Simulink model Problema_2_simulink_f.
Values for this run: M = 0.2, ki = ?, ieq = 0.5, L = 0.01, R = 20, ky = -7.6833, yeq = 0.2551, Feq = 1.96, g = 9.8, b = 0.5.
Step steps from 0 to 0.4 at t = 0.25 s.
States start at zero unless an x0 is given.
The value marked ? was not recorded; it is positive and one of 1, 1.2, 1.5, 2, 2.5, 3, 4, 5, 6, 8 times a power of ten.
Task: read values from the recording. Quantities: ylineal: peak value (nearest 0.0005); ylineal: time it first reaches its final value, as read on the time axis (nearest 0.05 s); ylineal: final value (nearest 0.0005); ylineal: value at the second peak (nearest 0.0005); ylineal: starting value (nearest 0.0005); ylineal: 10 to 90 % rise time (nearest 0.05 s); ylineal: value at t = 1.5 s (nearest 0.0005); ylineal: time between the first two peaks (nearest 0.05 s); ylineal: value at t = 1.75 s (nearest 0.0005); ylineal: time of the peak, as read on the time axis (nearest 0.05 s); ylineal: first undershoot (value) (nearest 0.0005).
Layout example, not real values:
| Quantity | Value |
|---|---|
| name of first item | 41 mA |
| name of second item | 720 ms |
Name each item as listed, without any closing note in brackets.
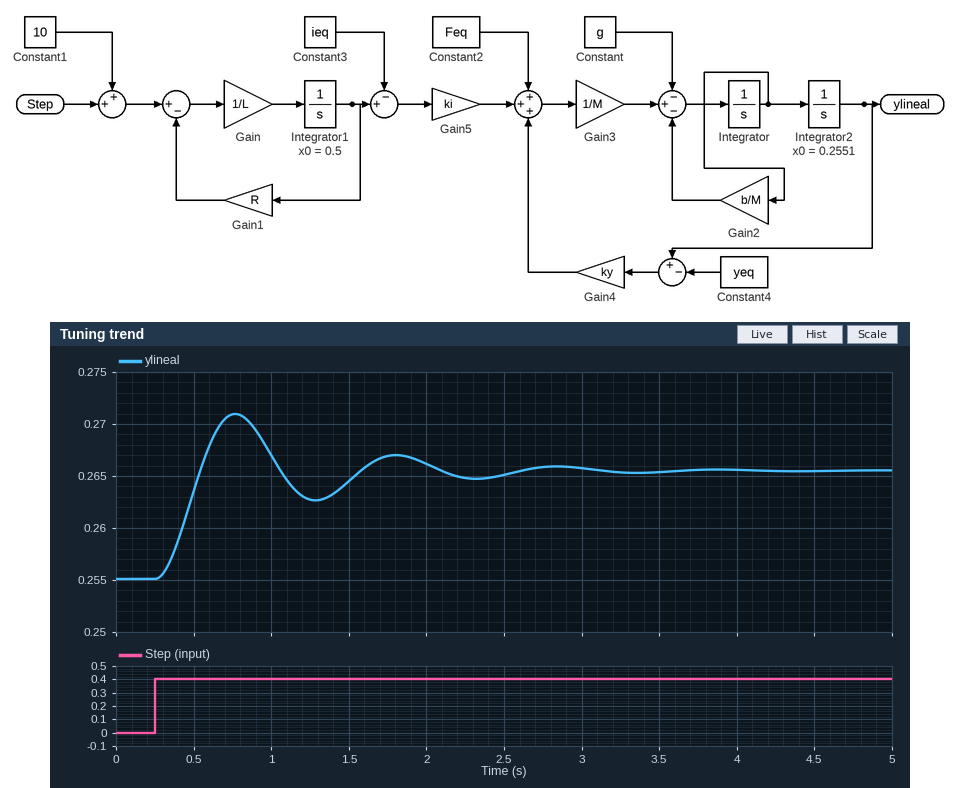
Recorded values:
| Quantity | Value |
|---|---|
| ylineal: peak value | 0.2710 |
| ylineal: time it first reaches its final value, as read on the time axis | 0.55 s |
| ylineal: final value | 0.2655 |
| ylineal: value at the second peak | 0.2670 |
| ylineal: starting value | 0.2550 |
| ylineal: 10 to 90 % rise time | 0.20 s |
| ylineal: value at t = 1.5 s | 0.2645 |
| ylineal: time between the first two peaks | 1.05 s |
| ylineal: value at t = 1.75 s | 0.2670 |
| ylineal: time of the peak, as read on the time axis | 0.75 s |
| ylineal: first undershoot (value) | 0.2625 |
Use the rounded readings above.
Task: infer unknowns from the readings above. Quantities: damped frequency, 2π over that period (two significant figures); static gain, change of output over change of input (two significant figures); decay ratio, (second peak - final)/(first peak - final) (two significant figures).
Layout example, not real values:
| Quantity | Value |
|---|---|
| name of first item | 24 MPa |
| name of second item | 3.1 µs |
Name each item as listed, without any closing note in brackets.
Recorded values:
| Quantity | Value |
|---|---|
| damped frequency, 2π over that period | 6.0 rad/s |
| static gain, change of output over change of input | 0.026 |
| decay ratio, (second peak - final)/(first peak - final) | 0.27 |
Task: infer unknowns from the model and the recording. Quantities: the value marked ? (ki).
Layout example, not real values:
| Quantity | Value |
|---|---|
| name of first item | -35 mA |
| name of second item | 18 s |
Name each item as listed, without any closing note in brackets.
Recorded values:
| Quantity | Value |
|---|---|
| the value marked ? | 4 |
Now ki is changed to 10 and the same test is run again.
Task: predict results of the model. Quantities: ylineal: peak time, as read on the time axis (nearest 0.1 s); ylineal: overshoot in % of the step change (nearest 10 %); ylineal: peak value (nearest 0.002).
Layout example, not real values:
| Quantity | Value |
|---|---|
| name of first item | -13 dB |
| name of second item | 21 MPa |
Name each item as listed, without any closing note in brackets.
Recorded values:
| Quantity | Value |
|---|---|
| ylineal: peak time, as read on the time axis | 0.8 s |
| ylineal: overshoot in % of the step change | 50 % |
| ylineal: peak value | 0.294 |
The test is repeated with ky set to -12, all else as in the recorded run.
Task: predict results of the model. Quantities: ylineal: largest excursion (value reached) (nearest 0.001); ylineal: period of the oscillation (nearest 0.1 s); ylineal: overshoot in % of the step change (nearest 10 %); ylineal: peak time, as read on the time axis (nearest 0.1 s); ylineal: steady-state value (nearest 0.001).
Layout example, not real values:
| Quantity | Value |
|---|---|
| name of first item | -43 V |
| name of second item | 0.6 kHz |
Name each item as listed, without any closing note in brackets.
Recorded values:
| Quantity | Value |
|---|---|
| ylineal: largest excursion (value reached) | 0.266 |
| ylineal: period of the oscillation | 0.8 s |
| ylineal: overshoot in % of the step change | 60 % |
| ylineal: peak time, as read on the time axis | 0.7 s |
| ylineal: steady-state value | 0.262 |
